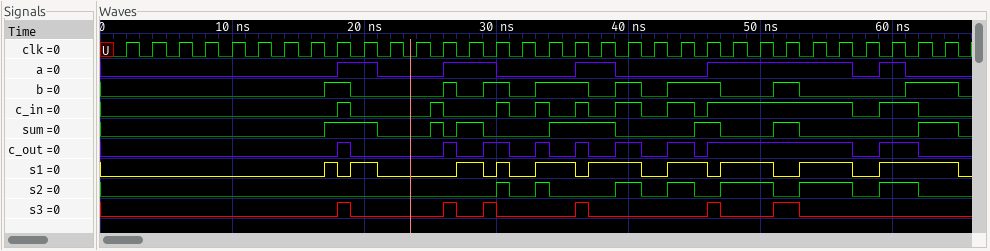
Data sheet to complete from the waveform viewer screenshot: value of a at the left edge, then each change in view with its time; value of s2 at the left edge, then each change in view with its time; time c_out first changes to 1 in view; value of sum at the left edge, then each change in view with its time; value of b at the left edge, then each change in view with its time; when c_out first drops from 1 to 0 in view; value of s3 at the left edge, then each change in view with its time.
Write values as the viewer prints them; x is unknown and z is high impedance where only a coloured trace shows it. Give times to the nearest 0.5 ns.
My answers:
0, 1 at 18 ns, 0 at 21 ns, 1 at 26 ns, 0 at 30 ns, 1 at 36 ns, 0 at 39 ns, 1 at 46 ns, 0 at 57 ns, 1 at 59 ns, 0 at 61 ns
0, 1 at 30 ns, 0 at 31 ns, 1 at 33 ns, 0 at 34 ns, 1 at 39 ns, 0 at 41 ns, 1 at 43 ns, 0 at 45 ns, 1 at 47 ns, 0 at 51 ns, 1 at 53 ns, 0 at 57 ns, 1 at 59 ns, 0 at 62 ns
18 ns
0, 1 at 17 ns, 0 at 21 ns, 1 at 25 ns, 0 at 26 ns, 1 at 27 ns, 0 at 29 ns, 1 at 34 ns, 0 at 39 ns, 1 at 45 ns, 0 at 47 ns, 1 at 51 ns, 0 at 53 ns, 1 at 62 ns, 0 at 65 ns
0, 1 at 17 ns, 0 at 19 ns, 1 at 26 ns, 0 at 27 ns, 1 at 29 ns, 0 at 31 ns, 1 at 33 ns, 0 at 37 ns, 1 at 39 ns, 0 at 41 ns, 1 at 43 ns, 0 at 47 ns, 1 at 51 ns, 0 at 53 ns, 1 at 61 ns, 0 at 65 ns
19 ns
0, 1 at 18 ns, 0 at 19 ns, 1 at 26 ns, 0 at 27 ns, 1 at 29 ns, 0 at 30 ns, 1 at 36 ns, 0 at 37 ns, 1 at 46 ns, 0 at 47 ns, 1 at 51 ns, 0 at 53 ns
